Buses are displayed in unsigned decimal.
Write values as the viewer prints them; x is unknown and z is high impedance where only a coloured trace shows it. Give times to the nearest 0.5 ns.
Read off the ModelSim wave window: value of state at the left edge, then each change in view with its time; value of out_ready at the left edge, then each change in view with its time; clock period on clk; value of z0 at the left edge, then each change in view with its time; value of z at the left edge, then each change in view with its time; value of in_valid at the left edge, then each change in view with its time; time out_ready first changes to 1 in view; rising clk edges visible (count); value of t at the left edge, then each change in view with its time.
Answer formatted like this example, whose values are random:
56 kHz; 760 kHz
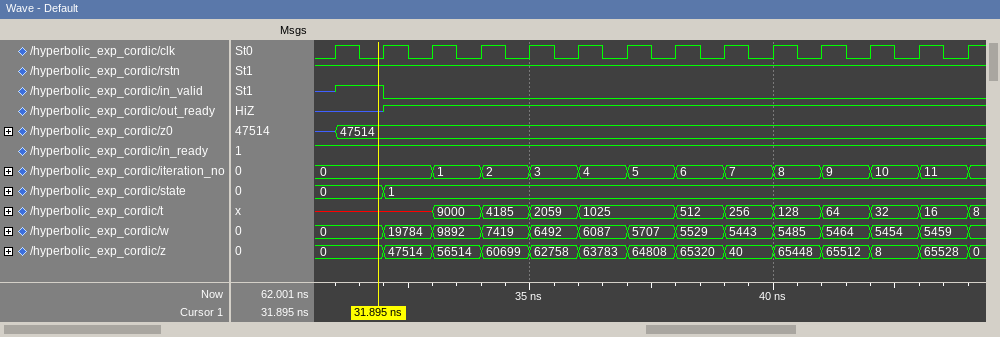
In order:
0, 1 at 32 ns; z, 1 at 32 ns; 1 ns; z, 47514 at 31 ns; 0, 47514 at 32 ns, 56514 at 33 ns, 60699 at 34 ns, 62758 at 35 ns, 63783 at 36 ns, 64808 at 37 ns, 65320 at 38 ns, 40 at 39 ns, 65448 at 40 ns, 65512 at 41 ns, 8 at 42 ns, 65528 at 43 ns, 0 at 44 ns; z, 1 at 31 ns, 0 at 32 ns; 32 ns; 14; x, 9000 at 33 ns, 4185 at 34 ns, 2059 at 35 ns, 1025 at 36 ns, 512 at 38 ns, 256 at 39 ns, 128 at 40 ns, 64 at 41 ns, 32 at 42 ns, 16 at 43 ns, 8 at 44 ns
